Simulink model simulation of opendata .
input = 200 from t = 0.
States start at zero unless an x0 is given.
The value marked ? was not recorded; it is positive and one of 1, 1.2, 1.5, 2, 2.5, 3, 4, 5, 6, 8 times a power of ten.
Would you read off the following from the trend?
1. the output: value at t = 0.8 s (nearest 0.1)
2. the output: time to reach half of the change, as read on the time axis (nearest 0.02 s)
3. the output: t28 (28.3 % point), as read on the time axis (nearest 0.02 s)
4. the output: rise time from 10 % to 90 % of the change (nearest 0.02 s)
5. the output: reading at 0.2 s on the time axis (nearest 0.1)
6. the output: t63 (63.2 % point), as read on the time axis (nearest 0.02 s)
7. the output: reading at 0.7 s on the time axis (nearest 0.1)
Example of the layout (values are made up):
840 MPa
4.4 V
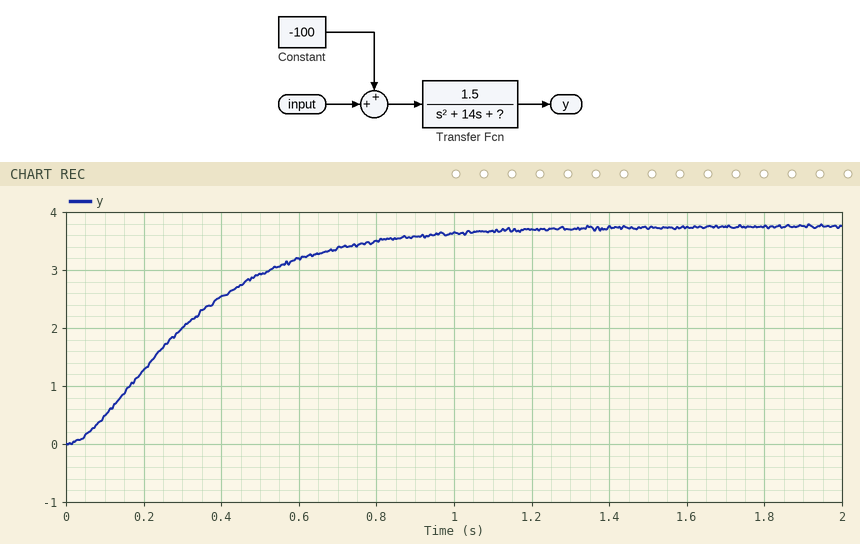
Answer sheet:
3.5
0.28 s
0.18 s
0.62 s
1.3
0.36 s
3.4
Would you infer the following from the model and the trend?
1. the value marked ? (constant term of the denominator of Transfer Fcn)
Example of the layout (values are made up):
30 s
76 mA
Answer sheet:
40
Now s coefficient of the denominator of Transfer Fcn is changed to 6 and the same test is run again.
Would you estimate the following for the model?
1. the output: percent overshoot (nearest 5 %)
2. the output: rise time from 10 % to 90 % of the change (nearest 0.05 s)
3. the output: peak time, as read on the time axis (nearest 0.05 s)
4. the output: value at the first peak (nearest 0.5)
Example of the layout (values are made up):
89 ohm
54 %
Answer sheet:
20 %
0.25 s
0.55 s
4.5
